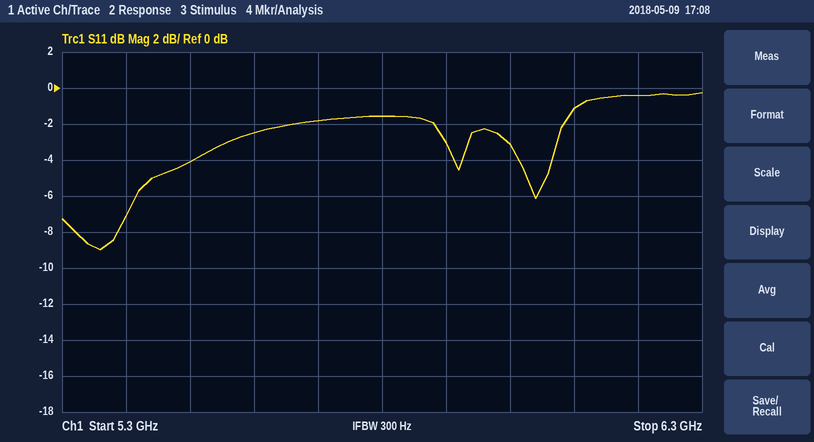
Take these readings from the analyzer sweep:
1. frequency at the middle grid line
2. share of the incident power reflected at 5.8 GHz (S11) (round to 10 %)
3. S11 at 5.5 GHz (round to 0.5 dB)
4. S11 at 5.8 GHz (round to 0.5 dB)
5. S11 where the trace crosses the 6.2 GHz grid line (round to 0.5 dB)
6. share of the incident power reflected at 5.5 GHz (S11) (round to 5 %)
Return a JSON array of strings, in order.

["5.8 GHz", "70 %", "-4.0 dB", "-1.5 dB", "-0.5 dB", "40 %"]
